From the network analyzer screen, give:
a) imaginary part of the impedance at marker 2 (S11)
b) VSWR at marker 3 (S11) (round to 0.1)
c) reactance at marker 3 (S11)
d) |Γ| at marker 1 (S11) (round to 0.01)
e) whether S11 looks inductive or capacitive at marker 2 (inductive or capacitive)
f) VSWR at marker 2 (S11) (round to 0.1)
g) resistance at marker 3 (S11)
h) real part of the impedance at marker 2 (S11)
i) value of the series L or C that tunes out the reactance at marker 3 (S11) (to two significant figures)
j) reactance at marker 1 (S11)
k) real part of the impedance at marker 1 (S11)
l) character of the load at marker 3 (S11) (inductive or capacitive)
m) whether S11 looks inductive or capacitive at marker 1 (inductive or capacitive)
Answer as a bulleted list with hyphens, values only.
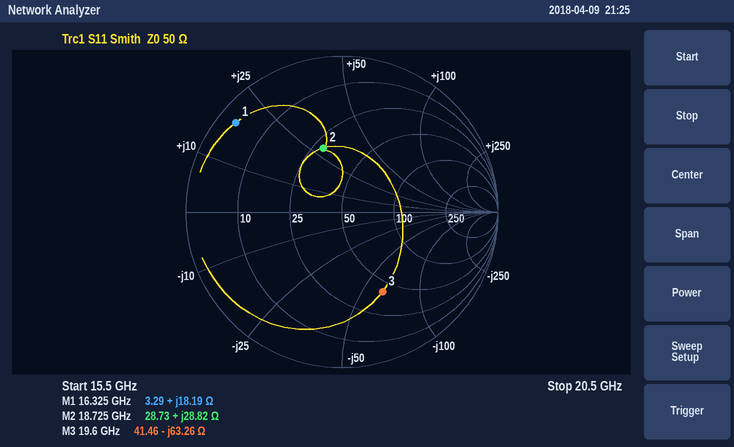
- +28.82 Ω
- 3.7
- -63.26 Ω
- 0.89
- inductive
- 2.5
- 41.46 Ω
- 28.73 Ω
- 510 pH
- +18.19 Ω
- 3.29 Ω
- capacitive
- inductive
